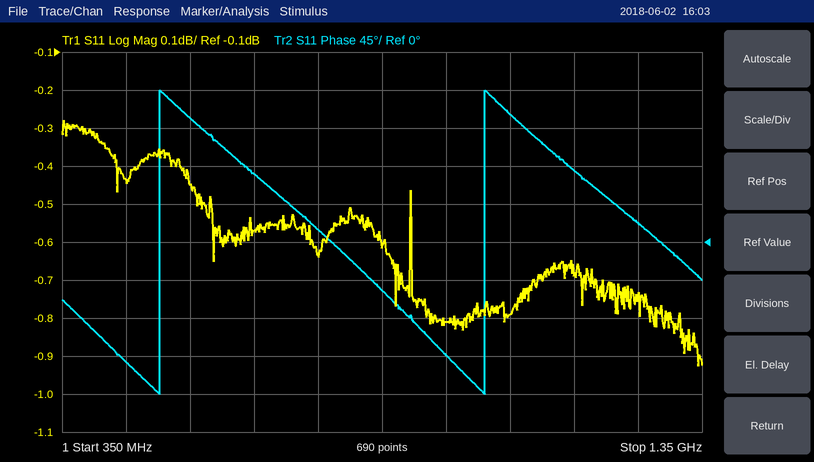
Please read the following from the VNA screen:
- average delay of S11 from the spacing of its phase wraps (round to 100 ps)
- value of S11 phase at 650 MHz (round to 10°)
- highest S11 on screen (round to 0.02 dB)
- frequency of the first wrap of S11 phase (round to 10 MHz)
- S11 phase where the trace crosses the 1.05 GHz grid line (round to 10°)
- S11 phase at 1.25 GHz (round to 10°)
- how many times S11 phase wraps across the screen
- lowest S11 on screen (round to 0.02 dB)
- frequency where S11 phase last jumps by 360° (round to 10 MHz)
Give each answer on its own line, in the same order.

2.0 ns
80°
-0.28 dB
500 MHz
150°
20°
2
-0.92 dB
1.01 GHz
